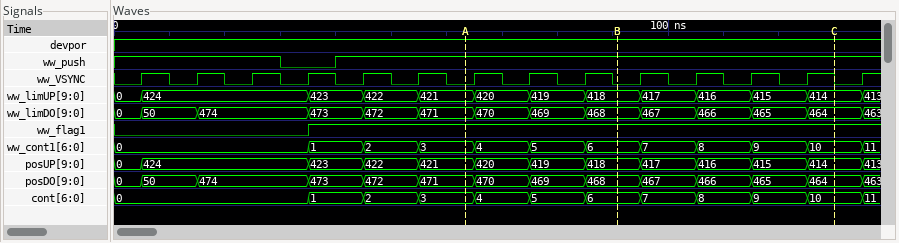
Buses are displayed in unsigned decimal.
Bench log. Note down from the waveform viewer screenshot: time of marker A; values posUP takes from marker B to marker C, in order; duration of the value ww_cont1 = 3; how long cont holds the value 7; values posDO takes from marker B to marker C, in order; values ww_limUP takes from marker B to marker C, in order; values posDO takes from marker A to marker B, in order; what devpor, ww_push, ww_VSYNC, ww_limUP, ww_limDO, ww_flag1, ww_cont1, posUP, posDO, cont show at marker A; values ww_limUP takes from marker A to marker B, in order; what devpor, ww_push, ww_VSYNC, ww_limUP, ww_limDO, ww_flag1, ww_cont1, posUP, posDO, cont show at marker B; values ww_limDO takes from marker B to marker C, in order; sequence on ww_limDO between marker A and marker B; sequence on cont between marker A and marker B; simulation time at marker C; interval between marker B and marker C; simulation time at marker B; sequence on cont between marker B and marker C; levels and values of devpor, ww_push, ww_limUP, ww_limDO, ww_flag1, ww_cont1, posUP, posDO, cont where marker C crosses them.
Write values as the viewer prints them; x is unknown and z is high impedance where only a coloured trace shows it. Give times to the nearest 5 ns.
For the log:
65 ns
418, 417, 416, 415, 414
10 ns
10 ns
468, 467, 466, 465, 464
418, 417, 416, 415, 414
471, 470, 469, 468
devpor=1, ww_push=1, ww_VSYNC=0, ww_limUP=421, ww_limDO=471, ww_flag1=1, ww_cont1=3, posUP=421, posDO=471, cont=3
421, 420, 419, 418
devpor=1, ww_push=1, ww_VSYNC=0, ww_limUP=418, ww_limDO=468, ww_flag1=1, ww_cont1=6, posUP=418, posDO=468, cont=6
468, 467, 466, 465, 464
471, 470, 469, 468
3, 4, 5, 6
130 ns
40 ns
90 ns
6, 7, 8, 9, 10
devpor=1, ww_push=1, ww_limUP=414, ww_limDO=464, ww_flag1=1, ww_cont1=10, posUP=414, posDO=464, cont=10
